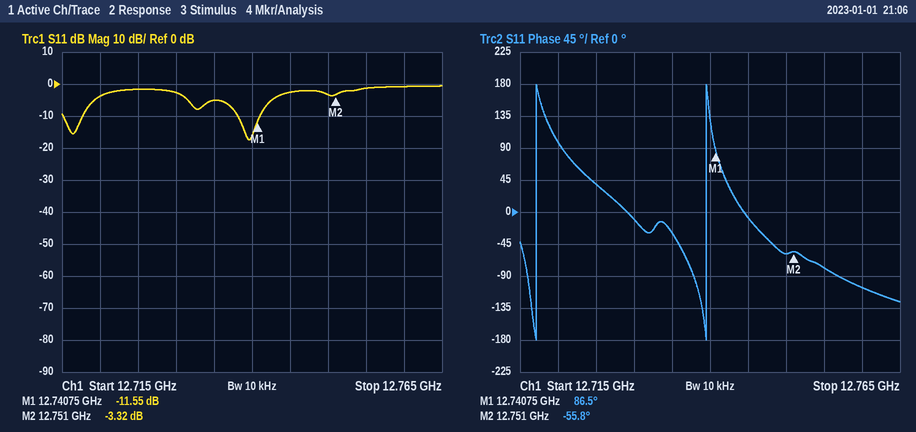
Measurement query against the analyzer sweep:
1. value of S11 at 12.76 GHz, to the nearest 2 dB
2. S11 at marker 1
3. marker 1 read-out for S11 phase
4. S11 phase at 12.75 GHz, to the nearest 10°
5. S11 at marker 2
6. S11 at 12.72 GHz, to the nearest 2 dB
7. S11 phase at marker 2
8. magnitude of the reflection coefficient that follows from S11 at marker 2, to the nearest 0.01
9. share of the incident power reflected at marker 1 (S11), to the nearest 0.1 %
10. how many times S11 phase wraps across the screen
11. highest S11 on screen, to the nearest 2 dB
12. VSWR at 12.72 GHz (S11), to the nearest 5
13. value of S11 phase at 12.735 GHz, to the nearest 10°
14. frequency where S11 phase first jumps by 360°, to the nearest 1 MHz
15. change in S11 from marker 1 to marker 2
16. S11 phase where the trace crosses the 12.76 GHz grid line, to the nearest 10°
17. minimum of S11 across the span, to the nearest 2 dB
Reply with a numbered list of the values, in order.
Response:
1. 0 dB
2. -11.55 dB
3. 86.5°
4. -60°
5. -3.32 dB
6. -4 dB
7. -55.8°
8. 0.68
9. 7.0 %
10. 2
11. 0 dB
12. 5
13. -30°
14. 12.717 GHz
15. 8.23 dB
16. -110°
17. -18 dB
